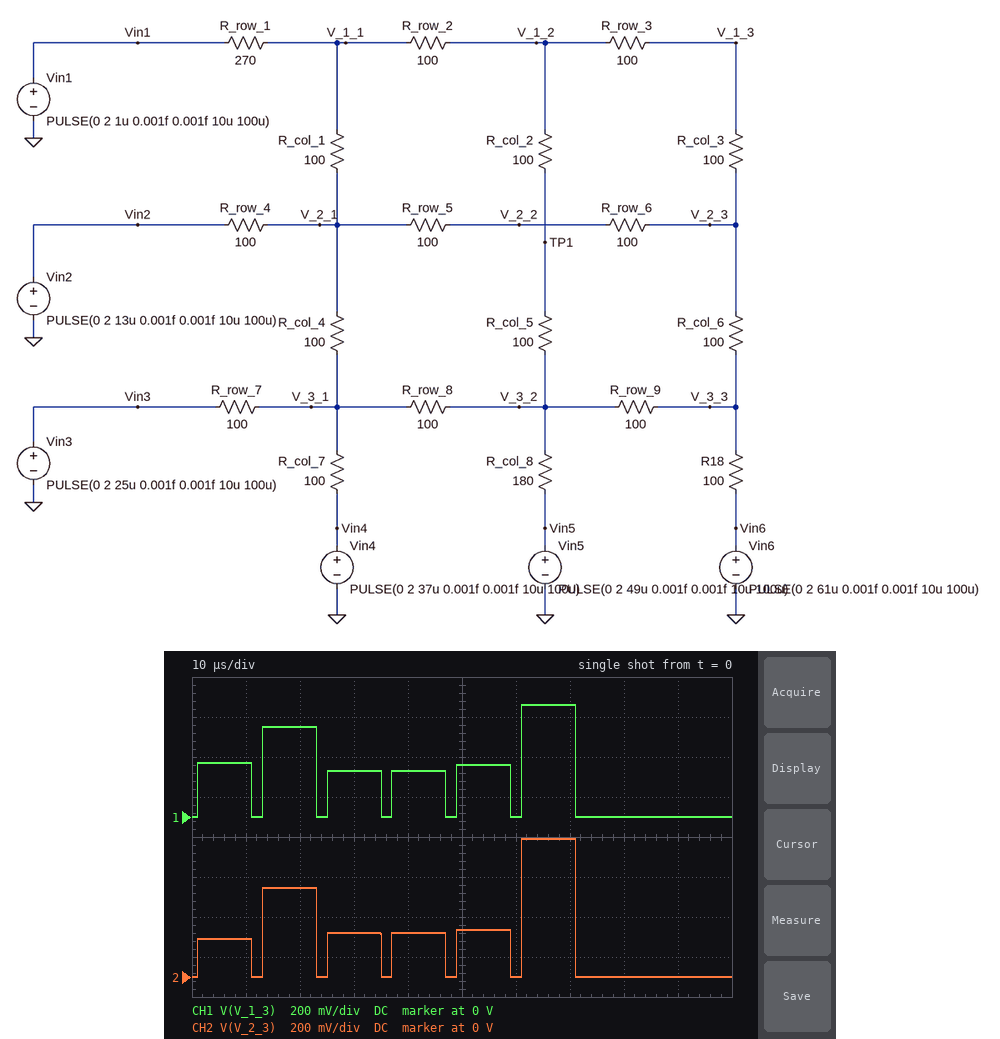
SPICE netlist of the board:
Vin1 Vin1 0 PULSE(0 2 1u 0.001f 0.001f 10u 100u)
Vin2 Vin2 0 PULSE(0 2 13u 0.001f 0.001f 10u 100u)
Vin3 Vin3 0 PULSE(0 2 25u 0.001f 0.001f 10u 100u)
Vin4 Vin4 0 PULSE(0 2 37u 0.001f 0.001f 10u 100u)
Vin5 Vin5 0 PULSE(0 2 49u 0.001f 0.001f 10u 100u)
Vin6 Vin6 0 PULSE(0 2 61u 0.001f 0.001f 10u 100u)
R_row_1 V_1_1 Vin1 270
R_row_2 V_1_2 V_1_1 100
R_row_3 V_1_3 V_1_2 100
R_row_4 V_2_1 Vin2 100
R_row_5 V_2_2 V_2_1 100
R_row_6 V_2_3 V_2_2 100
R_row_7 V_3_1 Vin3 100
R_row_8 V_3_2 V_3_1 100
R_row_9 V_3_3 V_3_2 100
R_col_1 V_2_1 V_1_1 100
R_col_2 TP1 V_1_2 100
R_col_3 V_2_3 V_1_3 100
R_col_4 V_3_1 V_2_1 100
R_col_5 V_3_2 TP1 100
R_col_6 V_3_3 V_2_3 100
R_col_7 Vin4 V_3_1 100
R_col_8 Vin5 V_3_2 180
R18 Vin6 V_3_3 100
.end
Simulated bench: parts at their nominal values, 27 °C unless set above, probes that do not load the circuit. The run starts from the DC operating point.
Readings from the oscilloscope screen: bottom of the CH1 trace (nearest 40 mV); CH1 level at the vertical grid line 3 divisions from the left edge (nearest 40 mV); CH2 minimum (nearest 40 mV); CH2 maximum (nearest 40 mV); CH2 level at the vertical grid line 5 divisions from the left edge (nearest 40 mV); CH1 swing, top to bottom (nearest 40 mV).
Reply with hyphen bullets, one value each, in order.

- 0 V
- 240 mV
- 0 V
- 680 mV
- 240 mV
- 560 mV
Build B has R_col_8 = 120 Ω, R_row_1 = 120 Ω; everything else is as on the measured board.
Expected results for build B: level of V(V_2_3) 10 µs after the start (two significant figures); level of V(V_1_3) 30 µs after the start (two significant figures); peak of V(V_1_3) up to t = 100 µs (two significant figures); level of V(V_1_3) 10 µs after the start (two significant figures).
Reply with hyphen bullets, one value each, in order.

- 310 mV
- 190 mV
- 500 mV
- 440 mV
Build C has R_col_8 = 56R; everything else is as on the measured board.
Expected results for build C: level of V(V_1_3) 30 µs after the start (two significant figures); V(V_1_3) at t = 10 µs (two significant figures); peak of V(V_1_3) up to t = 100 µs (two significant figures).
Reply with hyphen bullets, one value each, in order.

- 170 mV
- 250 mV
- 520 mV
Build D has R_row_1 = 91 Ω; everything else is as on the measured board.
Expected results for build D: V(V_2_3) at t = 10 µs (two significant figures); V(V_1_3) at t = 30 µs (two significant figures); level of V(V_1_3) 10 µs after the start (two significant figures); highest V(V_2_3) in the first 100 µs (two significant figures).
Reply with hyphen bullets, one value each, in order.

- 370 mV
- 190 mV
- 520 mV
- 660 mV
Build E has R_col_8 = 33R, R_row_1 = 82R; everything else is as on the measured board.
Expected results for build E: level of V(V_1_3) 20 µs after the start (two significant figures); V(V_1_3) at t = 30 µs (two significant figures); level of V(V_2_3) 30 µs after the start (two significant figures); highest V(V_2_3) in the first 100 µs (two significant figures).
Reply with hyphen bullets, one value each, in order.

- 300 mV
- 120 mV
- 130 mV
- 560 mV
